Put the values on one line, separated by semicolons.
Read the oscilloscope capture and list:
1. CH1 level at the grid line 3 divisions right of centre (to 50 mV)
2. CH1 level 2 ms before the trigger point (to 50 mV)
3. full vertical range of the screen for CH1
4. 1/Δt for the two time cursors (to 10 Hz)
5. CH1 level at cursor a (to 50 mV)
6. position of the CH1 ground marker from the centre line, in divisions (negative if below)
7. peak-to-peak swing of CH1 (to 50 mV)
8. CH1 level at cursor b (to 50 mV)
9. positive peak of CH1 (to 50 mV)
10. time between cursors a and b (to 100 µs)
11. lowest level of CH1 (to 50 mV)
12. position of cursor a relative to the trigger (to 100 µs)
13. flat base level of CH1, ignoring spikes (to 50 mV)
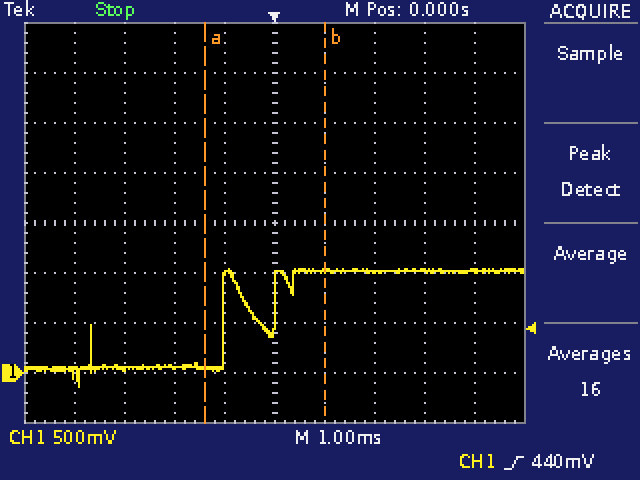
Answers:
1.00 V; 50 mV; 4 V; 420 Hz; 50 mV; -3.0 div; 1.20 V; 1.00 V; 1.05 V; 2.4 ms; -150 mV; -1.4 ms; 50 mV
